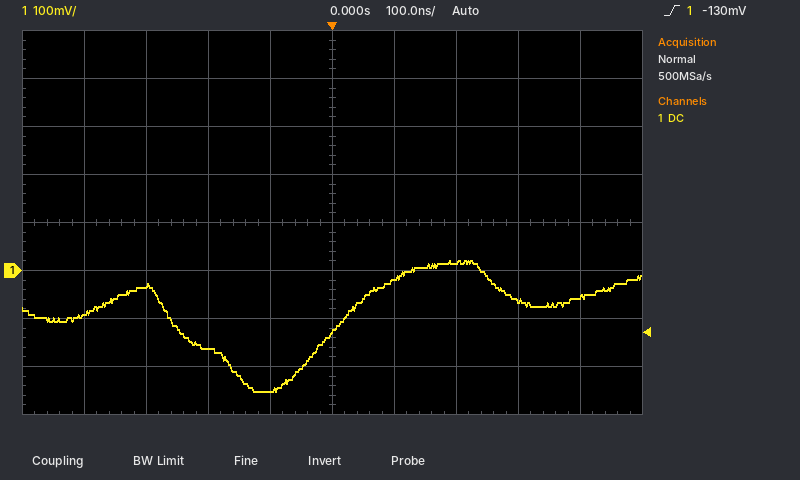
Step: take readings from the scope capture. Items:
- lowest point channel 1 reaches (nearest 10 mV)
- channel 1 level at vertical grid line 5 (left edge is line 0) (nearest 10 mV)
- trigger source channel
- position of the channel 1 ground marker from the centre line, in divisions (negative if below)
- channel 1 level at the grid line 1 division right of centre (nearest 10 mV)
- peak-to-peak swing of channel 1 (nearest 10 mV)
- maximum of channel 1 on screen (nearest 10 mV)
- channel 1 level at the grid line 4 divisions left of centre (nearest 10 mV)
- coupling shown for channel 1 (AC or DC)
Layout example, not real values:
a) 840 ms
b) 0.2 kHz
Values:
a) -250 mV
b) -130 mV
c) channel 1
d) -1.0 div
e) -20 mV
f) 270 mV
g) 20 mV
h) -90 mV
i) DC
